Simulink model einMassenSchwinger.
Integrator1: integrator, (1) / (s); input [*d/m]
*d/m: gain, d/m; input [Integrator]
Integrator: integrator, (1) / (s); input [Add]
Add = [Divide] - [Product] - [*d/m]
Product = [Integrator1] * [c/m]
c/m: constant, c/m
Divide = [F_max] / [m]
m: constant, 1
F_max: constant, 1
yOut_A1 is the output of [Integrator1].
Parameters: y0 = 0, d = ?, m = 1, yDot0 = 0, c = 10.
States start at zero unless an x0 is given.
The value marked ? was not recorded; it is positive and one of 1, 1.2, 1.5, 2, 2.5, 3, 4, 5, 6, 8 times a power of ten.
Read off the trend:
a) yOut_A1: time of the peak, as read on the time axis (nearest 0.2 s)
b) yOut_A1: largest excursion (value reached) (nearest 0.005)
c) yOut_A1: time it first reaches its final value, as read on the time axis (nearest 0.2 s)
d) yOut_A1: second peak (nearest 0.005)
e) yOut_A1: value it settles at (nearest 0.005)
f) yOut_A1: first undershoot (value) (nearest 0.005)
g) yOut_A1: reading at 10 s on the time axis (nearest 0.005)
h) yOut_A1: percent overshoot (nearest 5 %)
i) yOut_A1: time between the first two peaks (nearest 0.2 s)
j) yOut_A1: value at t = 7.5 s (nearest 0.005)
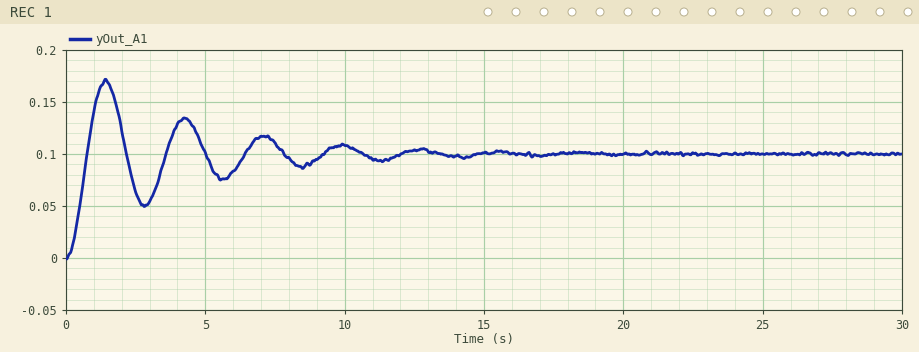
1.4 s
0.170
0.8 s
0.135
0.100
0.050
0.110
70 %
2.8 s
0.110
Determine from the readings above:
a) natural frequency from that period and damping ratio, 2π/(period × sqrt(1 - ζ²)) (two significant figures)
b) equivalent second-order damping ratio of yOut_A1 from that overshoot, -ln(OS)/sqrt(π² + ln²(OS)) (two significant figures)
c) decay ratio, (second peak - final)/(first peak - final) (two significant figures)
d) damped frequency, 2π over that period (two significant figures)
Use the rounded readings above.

2.3 rad/s
0.11
0.50
2.2 rad/s
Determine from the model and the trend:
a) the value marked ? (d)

0.5
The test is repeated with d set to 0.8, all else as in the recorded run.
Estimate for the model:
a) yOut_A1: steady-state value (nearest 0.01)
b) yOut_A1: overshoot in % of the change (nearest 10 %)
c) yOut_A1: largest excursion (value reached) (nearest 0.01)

0.10
60 %
0.16
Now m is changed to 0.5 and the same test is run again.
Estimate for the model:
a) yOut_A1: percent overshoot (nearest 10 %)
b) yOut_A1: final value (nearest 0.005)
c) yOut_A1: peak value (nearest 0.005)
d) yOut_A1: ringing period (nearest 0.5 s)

70 %
0.050
0.085
1.5 s
